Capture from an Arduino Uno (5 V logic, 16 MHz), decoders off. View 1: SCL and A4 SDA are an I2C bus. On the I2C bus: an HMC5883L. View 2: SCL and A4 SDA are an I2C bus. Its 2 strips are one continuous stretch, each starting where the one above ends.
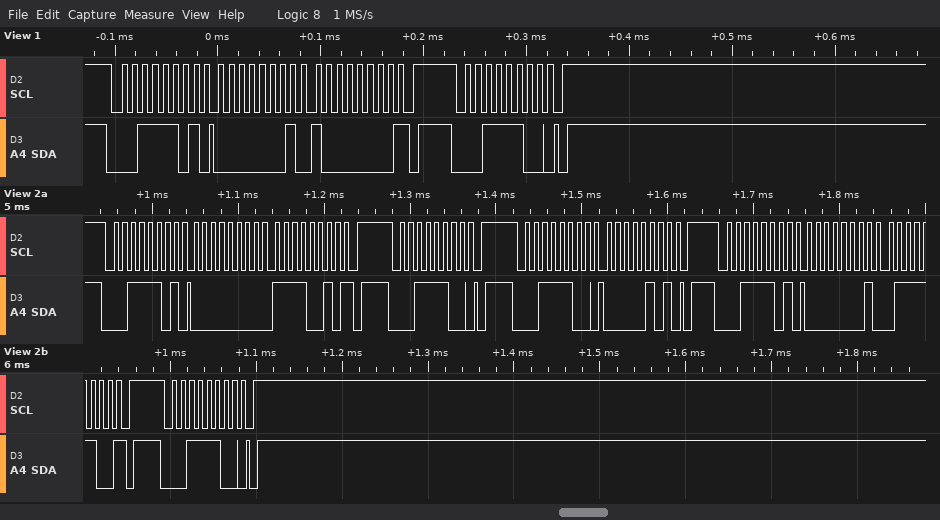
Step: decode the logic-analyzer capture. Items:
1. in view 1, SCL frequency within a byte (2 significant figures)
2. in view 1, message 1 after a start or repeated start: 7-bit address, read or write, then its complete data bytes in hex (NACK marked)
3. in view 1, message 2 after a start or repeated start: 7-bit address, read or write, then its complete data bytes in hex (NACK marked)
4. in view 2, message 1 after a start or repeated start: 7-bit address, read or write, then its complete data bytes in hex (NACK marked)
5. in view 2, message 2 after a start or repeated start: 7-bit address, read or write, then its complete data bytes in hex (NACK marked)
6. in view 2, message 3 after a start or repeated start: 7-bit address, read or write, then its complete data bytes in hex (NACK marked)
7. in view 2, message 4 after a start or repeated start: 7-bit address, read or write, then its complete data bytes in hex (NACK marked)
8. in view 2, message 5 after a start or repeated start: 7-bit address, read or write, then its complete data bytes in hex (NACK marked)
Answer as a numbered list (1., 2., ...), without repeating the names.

1. 100 kHz
2. 0x1E read: 01 80 NACK
3. 0x1E write
4. 0x1E read: 00 F2 NACK
5. 0x1E write
6. 0x1E write: 05
7. 0x1E read: 01 7C NACK
8. 0x1E write
